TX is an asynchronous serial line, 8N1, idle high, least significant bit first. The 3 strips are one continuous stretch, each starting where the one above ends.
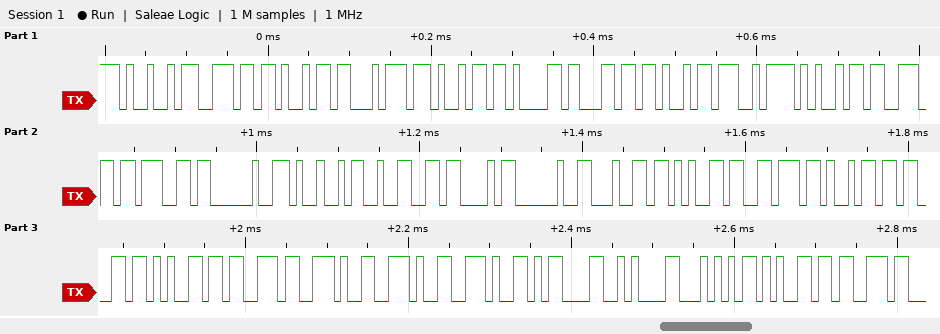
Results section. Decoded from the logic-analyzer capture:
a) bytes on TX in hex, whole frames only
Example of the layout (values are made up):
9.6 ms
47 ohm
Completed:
49 6E 69 74 69 61 6C 69 7A 69 6E 67 20 49 32 43 20 64 65 76 69 63 65 73 2E 2E 2E 0D 0A 54 65 73
